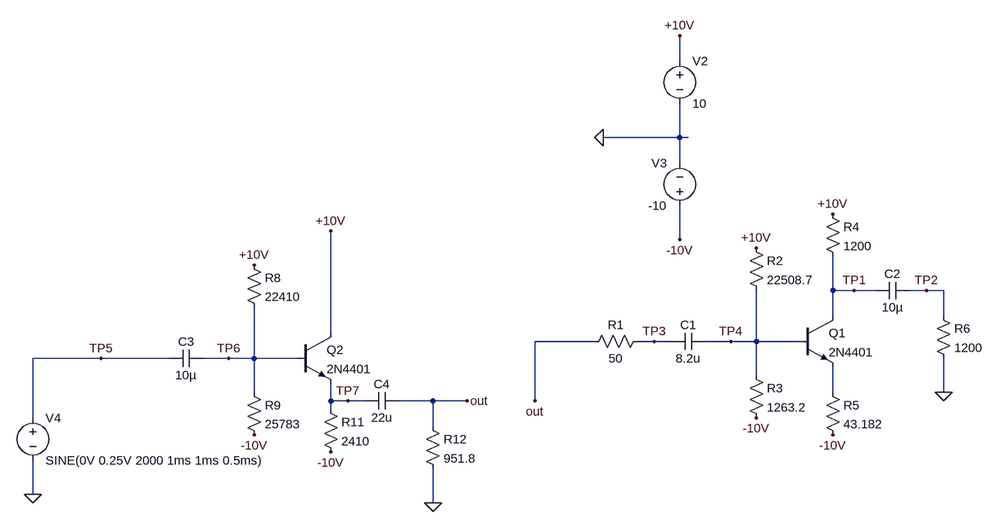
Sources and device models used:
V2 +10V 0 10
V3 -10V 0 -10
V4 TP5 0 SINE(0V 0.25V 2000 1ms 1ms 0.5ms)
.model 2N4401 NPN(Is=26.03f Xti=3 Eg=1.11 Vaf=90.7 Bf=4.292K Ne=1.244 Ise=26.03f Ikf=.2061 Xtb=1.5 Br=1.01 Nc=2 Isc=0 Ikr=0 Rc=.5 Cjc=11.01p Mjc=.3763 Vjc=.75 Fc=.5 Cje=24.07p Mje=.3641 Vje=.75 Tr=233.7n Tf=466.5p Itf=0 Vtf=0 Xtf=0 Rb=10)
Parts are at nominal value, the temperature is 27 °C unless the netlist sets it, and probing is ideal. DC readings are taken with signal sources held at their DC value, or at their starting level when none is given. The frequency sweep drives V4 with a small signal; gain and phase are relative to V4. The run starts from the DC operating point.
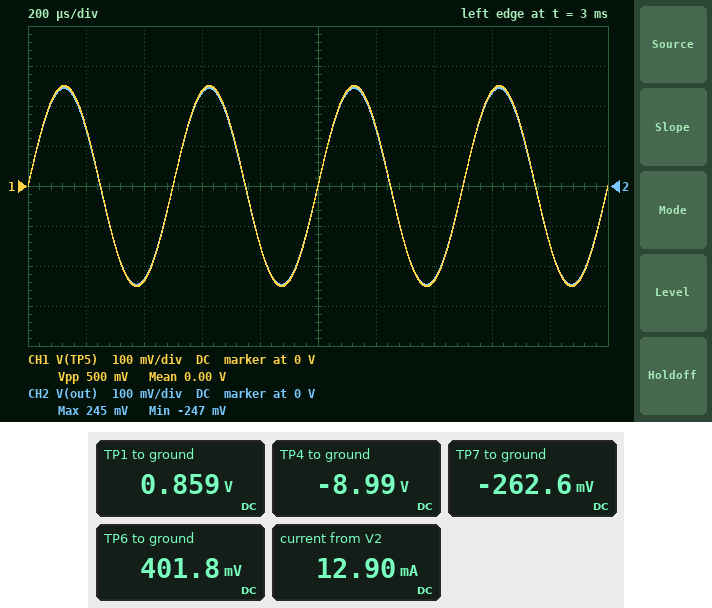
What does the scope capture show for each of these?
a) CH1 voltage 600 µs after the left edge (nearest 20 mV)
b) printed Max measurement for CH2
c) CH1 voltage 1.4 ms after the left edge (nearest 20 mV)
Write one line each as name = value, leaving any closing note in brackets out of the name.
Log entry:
CH1 voltage 600 µs after the left edge = 240 mV
printed Max measurement for CH2 = 245 mV
CH1 voltage 1.4 ms after the left edge = -240 mV
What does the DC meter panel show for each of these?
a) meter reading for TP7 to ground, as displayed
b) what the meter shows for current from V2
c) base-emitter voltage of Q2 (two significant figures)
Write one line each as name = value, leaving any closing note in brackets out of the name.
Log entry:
meter reading for TP7 to ground, as displayed = -262.6 mV
what the meter shows for current from V2 = 12.90 mA
base-emitter voltage of Q2 = 660 mV
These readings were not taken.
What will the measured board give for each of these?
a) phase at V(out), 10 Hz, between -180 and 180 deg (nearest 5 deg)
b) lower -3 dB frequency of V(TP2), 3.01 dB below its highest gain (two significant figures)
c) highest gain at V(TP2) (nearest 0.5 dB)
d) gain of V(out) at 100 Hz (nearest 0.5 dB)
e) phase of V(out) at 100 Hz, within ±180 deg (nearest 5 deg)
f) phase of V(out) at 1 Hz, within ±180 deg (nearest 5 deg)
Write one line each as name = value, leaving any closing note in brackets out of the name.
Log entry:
phase at V(out), 10 Hz, between -180 and 180 deg = 45 deg
lower -3 dB frequency of V(TP2), 3.01 dB below its highest gain = 29 Hz
highest gain at V(TP2) = 21.5 dB
gain of V(out) at 100 Hz = -0.5 dB
phase of V(out) at 100 Hz, within ±180 deg = 10 deg
phase of V(out) at 1 Hz, within ±180 deg = 135 deg
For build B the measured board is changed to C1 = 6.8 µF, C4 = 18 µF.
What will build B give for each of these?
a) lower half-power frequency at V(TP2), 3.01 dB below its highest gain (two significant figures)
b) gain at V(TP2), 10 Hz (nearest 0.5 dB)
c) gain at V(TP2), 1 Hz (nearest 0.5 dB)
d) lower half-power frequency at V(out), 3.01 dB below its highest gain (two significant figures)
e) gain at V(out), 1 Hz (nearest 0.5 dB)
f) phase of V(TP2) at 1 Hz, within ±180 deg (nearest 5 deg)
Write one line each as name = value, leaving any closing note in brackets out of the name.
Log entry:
lower half-power frequency at V(TP2), 3.01 dB below its highest gain = 34 Hz
gain at V(TP2), 10 Hz = 8.0 dB
gain at V(TP2), 1 Hz = -45.5 dB
lower half-power frequency at V(out), 3.01 dB below its highest gain = 18 Hz
gain at V(out), 1 Hz = -24.0 dB
phase of V(TP2) at 1 Hz, within ±180 deg = 125 deg
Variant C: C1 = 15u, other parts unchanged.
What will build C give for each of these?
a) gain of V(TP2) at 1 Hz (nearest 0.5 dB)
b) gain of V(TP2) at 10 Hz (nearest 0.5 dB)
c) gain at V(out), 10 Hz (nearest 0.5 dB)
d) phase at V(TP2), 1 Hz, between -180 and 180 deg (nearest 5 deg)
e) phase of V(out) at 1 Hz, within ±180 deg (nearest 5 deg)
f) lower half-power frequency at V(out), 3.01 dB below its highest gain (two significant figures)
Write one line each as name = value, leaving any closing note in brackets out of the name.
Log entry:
gain of V(TP2) at 1 Hz = -37.0 dB
gain of V(TP2) at 10 Hz = 12.5 dB
gain at V(out), 10 Hz = -5.0 dB
phase at V(TP2), 1 Hz, between -180 and 180 deg = 115 deg
phase of V(out) at 1 Hz, within ±180 deg = 130 deg
lower half-power frequency at V(out), 3.01 dB below its highest gain = 16 Hz
